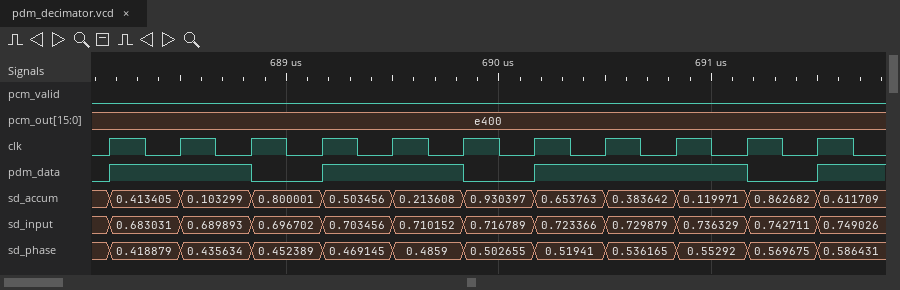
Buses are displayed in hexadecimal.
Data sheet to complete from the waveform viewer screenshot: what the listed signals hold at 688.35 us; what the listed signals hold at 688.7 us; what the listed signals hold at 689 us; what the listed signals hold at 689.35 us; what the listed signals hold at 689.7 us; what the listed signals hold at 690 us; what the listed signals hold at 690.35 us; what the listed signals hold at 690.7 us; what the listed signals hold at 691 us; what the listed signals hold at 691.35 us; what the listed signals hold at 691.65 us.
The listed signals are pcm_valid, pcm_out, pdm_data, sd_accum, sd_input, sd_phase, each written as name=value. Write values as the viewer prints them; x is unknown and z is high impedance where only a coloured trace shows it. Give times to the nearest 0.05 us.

pcm_valid=0, pcm_out=e400, pdm_data=1, sd_accum=0.413405, sd_input=0.683031, sd_phase=0.418879
pcm_valid=0, pcm_out=e400, pdm_data=1, sd_accum=0.103299, sd_input=0.689893, sd_phase=0.435634
pcm_valid=0, pcm_out=e400, pdm_data=0, sd_accum=0.800001, sd_input=0.696702, sd_phase=0.452389
pcm_valid=0, pcm_out=e400, pdm_data=1, sd_accum=0.503456, sd_input=0.703456, sd_phase=0.469145
pcm_valid=0, pcm_out=e400, pdm_data=1, sd_accum=0.213608, sd_input=0.710152, sd_phase=0.4859
pcm_valid=0, pcm_out=e400, pdm_data=0, sd_accum=0.930397, sd_input=0.716789, sd_phase=0.502655
pcm_valid=0, pcm_out=e400, pdm_data=1, sd_accum=0.653763, sd_input=0.723366, sd_phase=0.51941
pcm_valid=0, pcm_out=e400, pdm_data=1, sd_accum=0.383642, sd_input=0.729879, sd_phase=0.536165
pcm_valid=0, pcm_out=e400, pdm_data=1, sd_accum=0.119971, sd_input=0.736329, sd_phase=0.55292
pcm_valid=0, pcm_out=e400, pdm_data=0, sd_accum=0.862682, sd_input=0.742711, sd_phase=0.569675
pcm_valid=0, pcm_out=e400, pdm_data=1, sd_accum=0.611709, sd_input=0.749026, sd_phase=0.586431
